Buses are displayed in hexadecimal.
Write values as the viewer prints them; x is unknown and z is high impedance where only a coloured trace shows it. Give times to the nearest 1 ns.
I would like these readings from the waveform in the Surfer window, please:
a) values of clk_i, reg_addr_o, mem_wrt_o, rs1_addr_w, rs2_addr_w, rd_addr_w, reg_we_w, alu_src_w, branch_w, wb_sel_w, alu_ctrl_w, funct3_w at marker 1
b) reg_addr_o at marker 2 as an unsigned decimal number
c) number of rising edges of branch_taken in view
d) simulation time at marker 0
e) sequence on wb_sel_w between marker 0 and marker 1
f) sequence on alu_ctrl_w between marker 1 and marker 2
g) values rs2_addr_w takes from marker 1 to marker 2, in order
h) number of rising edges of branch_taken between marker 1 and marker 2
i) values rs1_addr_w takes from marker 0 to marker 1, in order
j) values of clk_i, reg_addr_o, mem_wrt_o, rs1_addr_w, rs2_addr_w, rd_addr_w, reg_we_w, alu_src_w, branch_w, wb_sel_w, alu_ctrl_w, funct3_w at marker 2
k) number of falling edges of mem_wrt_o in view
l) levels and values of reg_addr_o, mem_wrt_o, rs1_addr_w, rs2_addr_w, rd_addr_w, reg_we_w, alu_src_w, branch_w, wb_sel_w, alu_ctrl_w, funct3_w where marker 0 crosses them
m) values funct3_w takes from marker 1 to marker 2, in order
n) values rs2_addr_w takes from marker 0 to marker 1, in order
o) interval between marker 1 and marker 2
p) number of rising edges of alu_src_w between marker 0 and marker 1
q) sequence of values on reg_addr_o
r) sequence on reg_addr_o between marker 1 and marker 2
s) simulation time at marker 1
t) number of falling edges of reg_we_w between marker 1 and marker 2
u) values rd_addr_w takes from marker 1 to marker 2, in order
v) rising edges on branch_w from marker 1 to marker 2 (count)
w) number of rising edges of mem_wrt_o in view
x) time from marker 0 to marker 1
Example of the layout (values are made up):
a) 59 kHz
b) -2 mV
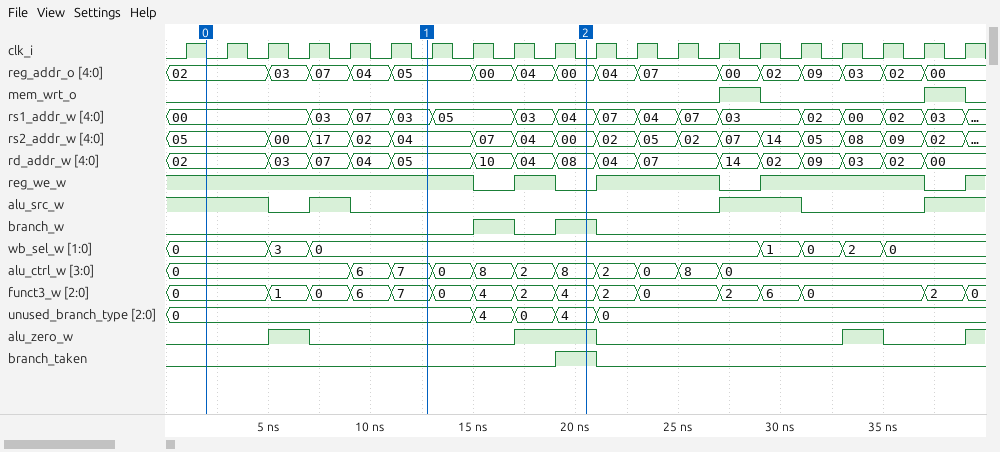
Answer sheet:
a) clk_i=0, reg_addr_o=05, mem_wrt_o=0, rs1_addr_w=03, rs2_addr_w=04, rd_addr_w=05, reg_we_w=1, alu_src_w=0, branch_w=0, wb_sel_w=0, alu_ctrl_w=7, funct3_w=7
b) 0
c) 1
d) 2 ns
e) 0, 3, 0
f) 7, 0, 8, 2, 8
g) 04, 07, 04, 00
h) 1
i) 00, 03, 07, 03
j) clk_i=0, reg_addr_o=00, mem_wrt_o=0, rs1_addr_w=04, rs2_addr_w=00, rd_addr_w=08, reg_we_w=0, alu_src_w=0, branch_w=1, wb_sel_w=0, alu_ctrl_w=8, funct3_w=4
k) 2
l) reg_addr_o=02, mem_wrt_o=0, rs1_addr_w=00, rs2_addr_w=05, rd_addr_w=02, reg_we_w=1, alu_src_w=1, branch_w=0, wb_sel_w=0, alu_ctrl_w=0, funct3_w=0
m) 7, 0, 4, 2, 4
n) 05, 00, 17, 02, 04
o) 8 ns
p) 1
q) 02, 03, 07, 04, 05, 00, 04, 00, 04, 07, 00, 02, 09, 03, 02, 00
r) 05, 00, 04, 00
s) 13 ns
t) 2
u) 05, 10, 04, 08
v) 2
w) 2
x) 11 ns
